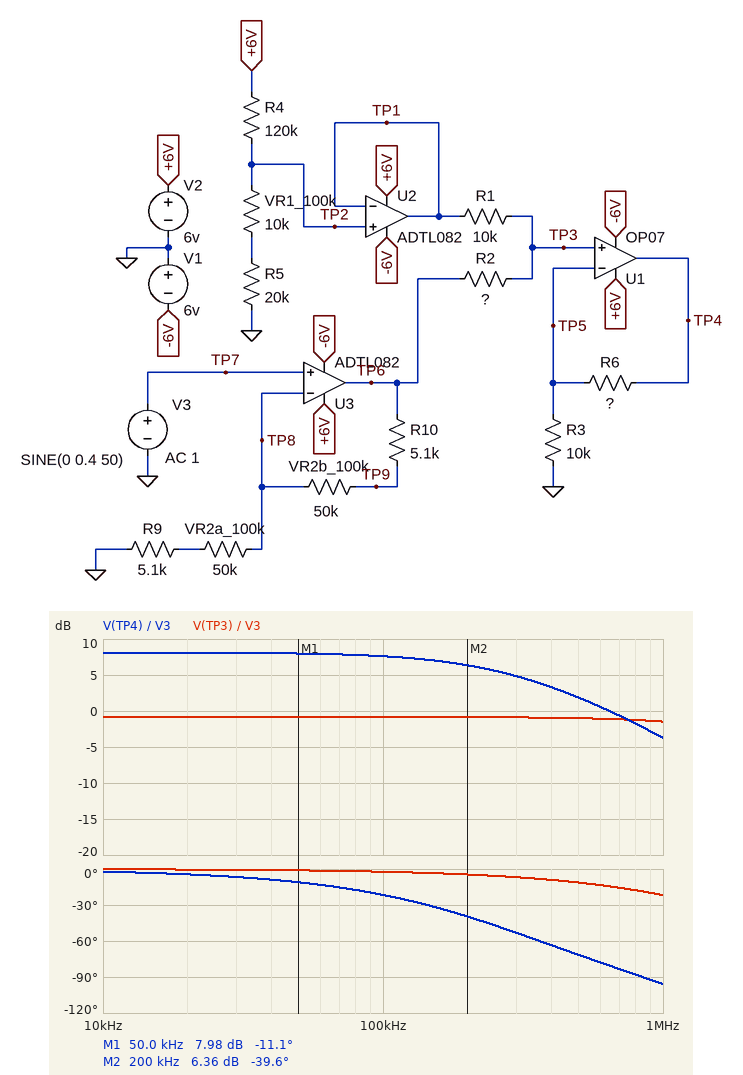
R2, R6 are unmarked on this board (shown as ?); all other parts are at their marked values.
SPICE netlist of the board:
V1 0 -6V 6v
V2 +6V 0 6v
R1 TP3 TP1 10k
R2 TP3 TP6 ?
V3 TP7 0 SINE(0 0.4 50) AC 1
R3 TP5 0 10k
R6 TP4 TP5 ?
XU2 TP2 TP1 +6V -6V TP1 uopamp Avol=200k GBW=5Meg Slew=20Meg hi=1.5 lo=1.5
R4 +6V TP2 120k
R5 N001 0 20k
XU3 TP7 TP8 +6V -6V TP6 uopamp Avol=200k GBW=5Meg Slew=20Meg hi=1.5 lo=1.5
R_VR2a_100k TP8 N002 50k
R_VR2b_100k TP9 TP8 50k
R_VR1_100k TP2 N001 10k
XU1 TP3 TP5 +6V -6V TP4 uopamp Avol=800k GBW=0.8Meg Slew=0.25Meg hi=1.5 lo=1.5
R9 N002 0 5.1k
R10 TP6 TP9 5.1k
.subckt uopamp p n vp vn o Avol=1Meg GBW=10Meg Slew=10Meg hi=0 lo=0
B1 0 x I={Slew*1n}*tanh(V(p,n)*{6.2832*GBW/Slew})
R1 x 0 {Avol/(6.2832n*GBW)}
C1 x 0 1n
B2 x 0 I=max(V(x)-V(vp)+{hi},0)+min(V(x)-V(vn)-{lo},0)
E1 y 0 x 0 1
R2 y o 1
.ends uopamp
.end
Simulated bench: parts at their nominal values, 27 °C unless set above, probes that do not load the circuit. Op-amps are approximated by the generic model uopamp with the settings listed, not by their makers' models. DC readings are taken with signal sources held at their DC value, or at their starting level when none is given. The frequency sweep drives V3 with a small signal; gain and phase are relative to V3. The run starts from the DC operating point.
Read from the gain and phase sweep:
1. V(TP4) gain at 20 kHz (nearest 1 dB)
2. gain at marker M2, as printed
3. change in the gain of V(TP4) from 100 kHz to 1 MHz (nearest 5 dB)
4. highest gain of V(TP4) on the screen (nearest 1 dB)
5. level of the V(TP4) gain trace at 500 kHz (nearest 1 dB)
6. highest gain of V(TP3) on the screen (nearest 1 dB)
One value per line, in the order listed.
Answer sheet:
8 dB
6.36 dB
-10 dB
8 dB
2 dB
-1 dB
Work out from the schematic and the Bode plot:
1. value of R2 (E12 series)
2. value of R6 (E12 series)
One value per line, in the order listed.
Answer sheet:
12 kΩ
18 kΩ
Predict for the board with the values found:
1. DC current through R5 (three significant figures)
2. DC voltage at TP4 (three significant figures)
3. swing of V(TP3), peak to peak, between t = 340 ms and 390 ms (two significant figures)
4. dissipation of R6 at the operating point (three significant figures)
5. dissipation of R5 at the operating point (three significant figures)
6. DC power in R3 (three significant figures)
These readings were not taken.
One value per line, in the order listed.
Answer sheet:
40.0 µA
1.83 V
730 mV
77.1 µW
32.0 µW
42.8 µW
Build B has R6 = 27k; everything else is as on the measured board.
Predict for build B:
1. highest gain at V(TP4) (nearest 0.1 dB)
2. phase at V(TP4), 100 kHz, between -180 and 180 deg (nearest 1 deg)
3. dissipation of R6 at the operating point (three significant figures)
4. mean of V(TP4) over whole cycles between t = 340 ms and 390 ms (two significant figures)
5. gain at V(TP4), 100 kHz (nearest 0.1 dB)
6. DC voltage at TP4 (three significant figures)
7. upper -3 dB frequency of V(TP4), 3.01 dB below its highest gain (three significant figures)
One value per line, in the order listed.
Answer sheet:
10.5 dB
-27 deg
116 µW
2.4 V
9.7 dB
2.42 V
215 kHz
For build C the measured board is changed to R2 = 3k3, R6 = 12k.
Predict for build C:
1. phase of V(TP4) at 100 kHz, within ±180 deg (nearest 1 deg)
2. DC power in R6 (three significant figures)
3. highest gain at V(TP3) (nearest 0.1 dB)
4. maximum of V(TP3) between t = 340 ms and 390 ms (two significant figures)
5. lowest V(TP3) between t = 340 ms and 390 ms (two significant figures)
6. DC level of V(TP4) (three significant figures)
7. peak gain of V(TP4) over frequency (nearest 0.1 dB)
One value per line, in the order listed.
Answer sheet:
-18 deg
10.6 µW
3.5 dB
900 mV
-300 mV
655 mV
10.4 dB
